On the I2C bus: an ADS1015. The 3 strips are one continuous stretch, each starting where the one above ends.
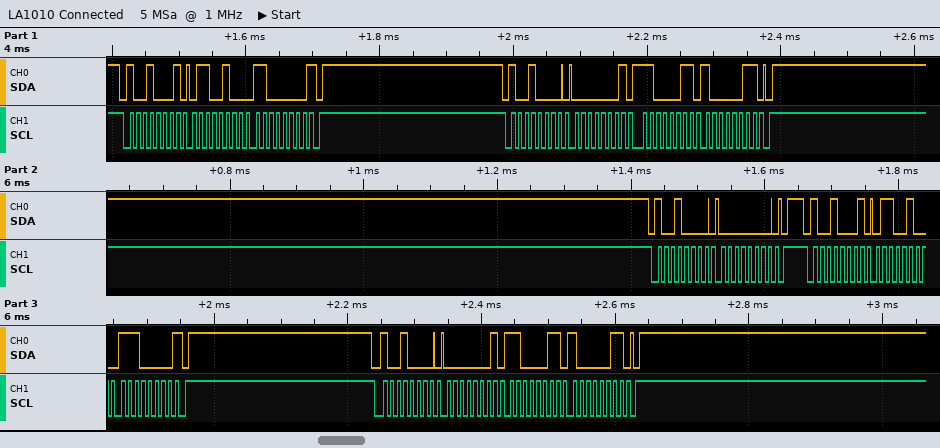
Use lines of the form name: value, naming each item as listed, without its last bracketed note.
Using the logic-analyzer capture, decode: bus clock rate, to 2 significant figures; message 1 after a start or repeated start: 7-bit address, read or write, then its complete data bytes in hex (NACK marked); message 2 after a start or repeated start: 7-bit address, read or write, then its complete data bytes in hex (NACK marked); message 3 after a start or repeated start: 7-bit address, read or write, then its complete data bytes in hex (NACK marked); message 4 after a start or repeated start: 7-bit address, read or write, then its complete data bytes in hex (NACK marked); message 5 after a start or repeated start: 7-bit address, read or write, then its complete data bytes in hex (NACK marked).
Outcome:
bus clock rate, to 2 significant figures: 100 kHz
message 1 after a start or repeated start: 7-bit address, read or write, then its complete data bytes in hex: 0x48 read: 64 C0 NACK
message 2 after a start or repeated start: 7-bit address, read or write, then its complete data bytes in hex: 0x48 write: 01 C3 83
message 3 after a start or repeated start: 7-bit address, read or write, then its complete data bytes in hex: 0x48 write: 00
message 4 after a start or repeated start: 7-bit address, read or write, then its complete data bytes in hex: 0x48 read: 64 E0 NACK
message 5 after a start or repeated start: 7-bit address, read or write, then its complete data bytes in hex: 0x48 write: 01 C3 83
